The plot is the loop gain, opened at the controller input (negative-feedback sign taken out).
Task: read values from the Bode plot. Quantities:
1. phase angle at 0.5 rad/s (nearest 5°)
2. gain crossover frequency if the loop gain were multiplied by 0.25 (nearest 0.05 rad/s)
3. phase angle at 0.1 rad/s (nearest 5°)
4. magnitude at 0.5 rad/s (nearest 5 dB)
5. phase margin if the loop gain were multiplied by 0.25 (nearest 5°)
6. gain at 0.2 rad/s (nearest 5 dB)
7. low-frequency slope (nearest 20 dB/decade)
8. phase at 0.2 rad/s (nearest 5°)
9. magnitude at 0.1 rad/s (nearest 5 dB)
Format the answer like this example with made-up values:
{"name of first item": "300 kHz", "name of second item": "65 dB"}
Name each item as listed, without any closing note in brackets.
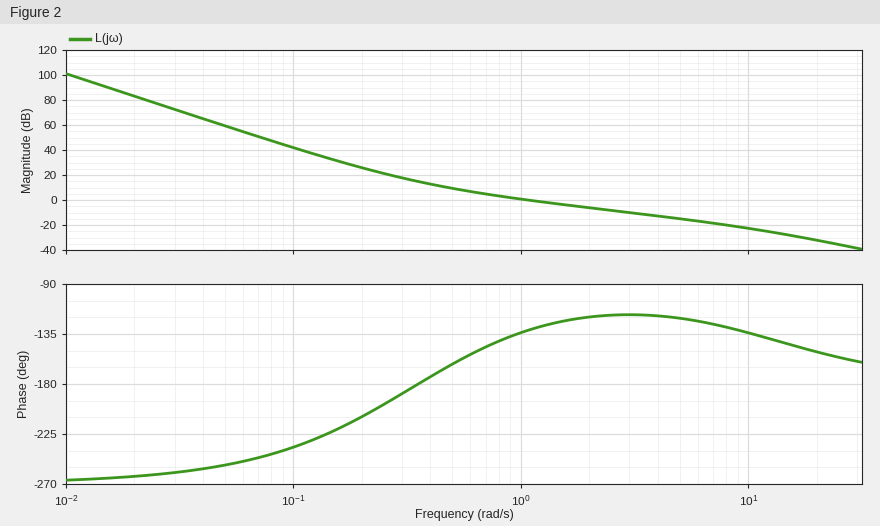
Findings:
{"phase angle at 0.5 rad/s": "-160°", "gain crossover frequency if the loop gain were multiplied by 0.25": "0.40 rad/s", "phase angle at 0.1 rad/s": "-235°", "magnitude at 0.5 rad/s": "10 dB", "phase margin if the loop gain were multiplied by 0.25": "10°", "gain at 0.2 rad/s": "25 dB", "low-frequency slope": "-60 dB/decade", "phase at 0.2 rad/s": "-210°", "magnitude at 0.1 rad/s": "40 dB"}
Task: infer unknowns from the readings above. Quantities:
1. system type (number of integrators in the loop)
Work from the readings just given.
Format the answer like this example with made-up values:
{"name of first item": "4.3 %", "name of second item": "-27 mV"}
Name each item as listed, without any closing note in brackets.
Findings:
{"system type": "3"}
